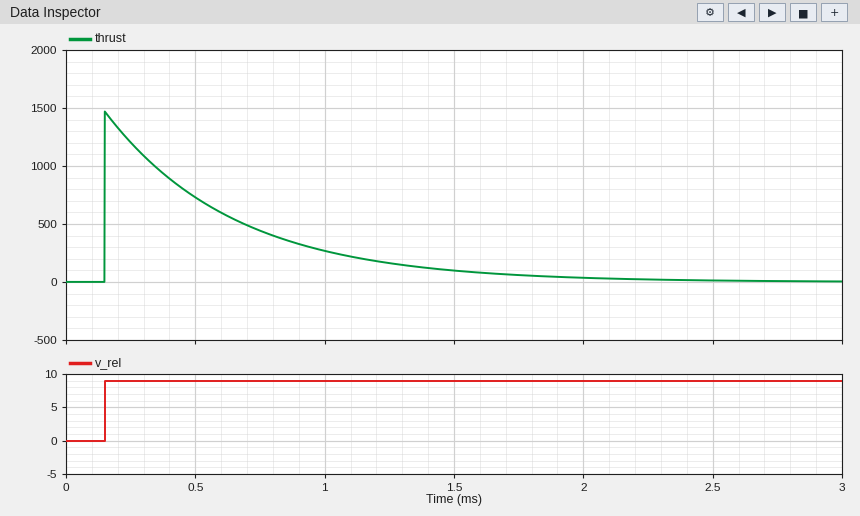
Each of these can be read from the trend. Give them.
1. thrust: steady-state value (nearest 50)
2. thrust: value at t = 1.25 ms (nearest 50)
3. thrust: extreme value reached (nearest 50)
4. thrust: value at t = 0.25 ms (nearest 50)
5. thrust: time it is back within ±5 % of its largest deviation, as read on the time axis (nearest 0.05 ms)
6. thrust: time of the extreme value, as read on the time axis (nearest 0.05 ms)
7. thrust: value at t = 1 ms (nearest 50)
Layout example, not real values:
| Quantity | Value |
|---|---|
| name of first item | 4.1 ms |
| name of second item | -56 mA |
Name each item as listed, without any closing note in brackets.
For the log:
| Quantity | Value |
|---|---|
| thrust: steady-state value | 0 |
| thrust: value at t = 1.25 ms | 150 |
| thrust: extreme value reached | 1450 |
| thrust: value at t = 0.25 ms | 1200 |
| thrust: time it is back within ±5 % of its largest deviation, as read on the time axis | 1.65 ms |
| thrust: time of the extreme value, as read on the time axis | 0.15 ms |
| thrust: value at t = 1 ms | 250 |
